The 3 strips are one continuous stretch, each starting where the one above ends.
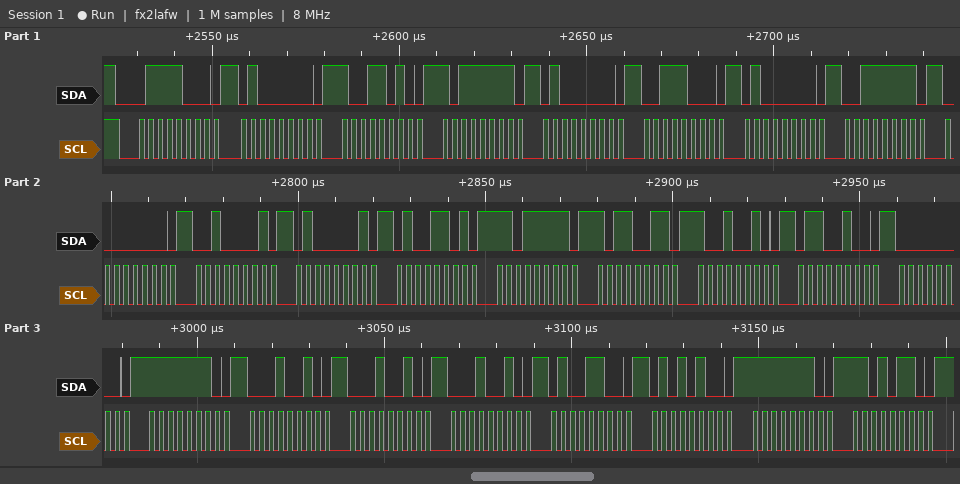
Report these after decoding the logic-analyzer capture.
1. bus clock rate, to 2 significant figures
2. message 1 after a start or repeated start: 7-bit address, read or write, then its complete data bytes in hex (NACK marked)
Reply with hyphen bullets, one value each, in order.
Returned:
- 400 kHz
- 0x3C write: 40 9A BF 40 38 40 3F 00 21 41 4D DF B3 92 64 00 FE 12 12 12 4C 54 FE D6
